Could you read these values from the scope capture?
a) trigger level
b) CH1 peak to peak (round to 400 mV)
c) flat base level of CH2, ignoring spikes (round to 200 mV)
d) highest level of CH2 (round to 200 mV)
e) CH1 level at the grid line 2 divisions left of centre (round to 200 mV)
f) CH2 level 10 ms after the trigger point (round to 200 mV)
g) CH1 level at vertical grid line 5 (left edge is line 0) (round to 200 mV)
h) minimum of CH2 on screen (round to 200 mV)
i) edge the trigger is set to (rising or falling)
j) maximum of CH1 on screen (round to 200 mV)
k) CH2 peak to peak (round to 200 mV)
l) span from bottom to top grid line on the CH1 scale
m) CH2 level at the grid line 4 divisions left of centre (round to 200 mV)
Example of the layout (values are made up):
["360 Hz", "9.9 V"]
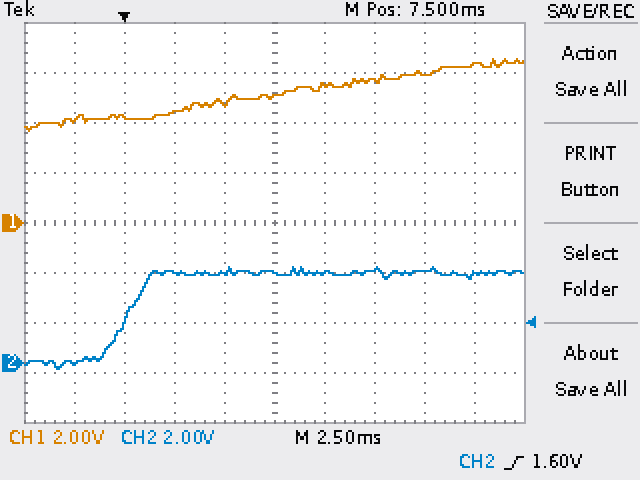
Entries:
["1.60 V", "2.8 V", "0.0 V", "3.8 V", "4.4 V", "3.6 V", "5.0 V", "-200 mV", "rising", "6.6 V", "4.0 V", "16 V", "0.0 V"]
